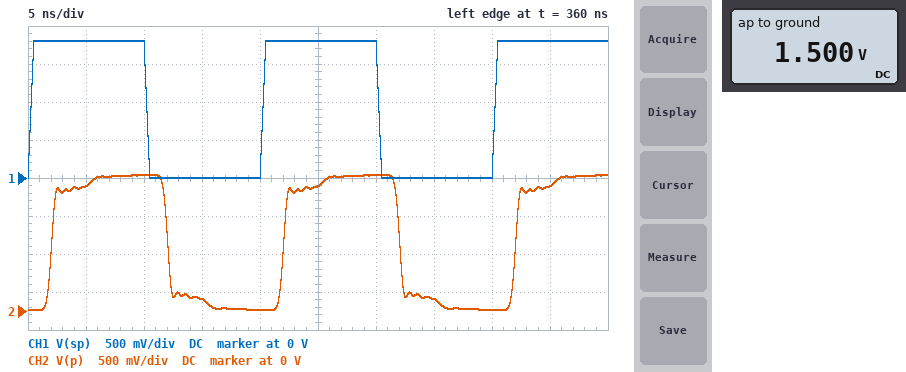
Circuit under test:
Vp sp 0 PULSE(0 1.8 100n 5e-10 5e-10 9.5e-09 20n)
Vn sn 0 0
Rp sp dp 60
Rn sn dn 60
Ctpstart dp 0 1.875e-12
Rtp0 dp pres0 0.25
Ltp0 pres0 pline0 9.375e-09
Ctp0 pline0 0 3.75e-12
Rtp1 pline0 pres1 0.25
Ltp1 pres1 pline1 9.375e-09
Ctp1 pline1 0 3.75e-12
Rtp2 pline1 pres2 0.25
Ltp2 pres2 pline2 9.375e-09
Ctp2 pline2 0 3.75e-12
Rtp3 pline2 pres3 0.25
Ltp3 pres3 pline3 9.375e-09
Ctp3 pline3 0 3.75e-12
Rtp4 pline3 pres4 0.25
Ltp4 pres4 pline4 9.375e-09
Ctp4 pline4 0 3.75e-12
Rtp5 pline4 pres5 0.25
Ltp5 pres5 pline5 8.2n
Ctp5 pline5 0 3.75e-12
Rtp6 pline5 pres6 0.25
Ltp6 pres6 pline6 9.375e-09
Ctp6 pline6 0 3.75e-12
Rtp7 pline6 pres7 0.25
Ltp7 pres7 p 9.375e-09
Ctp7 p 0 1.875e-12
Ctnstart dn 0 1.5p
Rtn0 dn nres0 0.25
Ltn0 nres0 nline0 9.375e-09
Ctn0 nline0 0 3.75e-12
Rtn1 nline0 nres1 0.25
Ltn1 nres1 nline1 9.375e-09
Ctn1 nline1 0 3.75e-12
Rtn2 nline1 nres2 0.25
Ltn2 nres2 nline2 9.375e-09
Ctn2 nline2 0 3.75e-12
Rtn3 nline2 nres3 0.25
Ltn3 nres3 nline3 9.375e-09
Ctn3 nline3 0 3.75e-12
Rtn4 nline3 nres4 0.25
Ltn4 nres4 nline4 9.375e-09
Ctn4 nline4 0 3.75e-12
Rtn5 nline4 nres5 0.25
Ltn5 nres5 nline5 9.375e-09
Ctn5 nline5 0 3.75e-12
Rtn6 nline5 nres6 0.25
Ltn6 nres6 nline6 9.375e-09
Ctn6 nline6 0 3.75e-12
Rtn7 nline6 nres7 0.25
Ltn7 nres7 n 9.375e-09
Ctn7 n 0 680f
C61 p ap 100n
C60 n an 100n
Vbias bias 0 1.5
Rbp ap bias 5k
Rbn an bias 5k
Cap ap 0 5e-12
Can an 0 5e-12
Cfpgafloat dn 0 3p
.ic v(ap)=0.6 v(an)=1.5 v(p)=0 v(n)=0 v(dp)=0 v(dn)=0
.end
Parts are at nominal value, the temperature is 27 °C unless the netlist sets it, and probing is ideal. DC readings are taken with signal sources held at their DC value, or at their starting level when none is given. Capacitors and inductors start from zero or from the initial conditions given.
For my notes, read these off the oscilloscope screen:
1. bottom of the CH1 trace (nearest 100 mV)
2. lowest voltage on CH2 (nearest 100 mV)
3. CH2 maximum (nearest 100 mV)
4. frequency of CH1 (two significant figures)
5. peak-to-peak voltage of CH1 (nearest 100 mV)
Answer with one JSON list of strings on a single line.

["0 V", "0 V", "1.8 V", "50 MHz", "1.8 V"]
